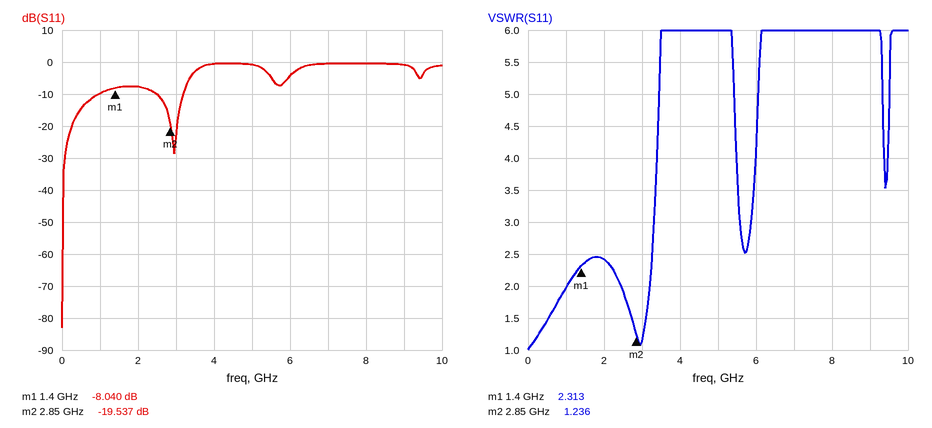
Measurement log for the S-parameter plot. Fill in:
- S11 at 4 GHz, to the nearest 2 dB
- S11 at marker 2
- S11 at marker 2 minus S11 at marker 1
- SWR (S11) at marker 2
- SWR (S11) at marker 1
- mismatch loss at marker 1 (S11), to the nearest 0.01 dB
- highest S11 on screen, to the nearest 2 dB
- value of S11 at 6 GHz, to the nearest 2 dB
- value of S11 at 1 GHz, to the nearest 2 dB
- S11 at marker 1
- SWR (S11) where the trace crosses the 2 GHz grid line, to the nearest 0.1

0 dB
-19.537 dB
-11.497 dB
1.236
2.313
0.74 dB
0 dB
-4 dB
-10 dB
-8.040 dB
2.4
